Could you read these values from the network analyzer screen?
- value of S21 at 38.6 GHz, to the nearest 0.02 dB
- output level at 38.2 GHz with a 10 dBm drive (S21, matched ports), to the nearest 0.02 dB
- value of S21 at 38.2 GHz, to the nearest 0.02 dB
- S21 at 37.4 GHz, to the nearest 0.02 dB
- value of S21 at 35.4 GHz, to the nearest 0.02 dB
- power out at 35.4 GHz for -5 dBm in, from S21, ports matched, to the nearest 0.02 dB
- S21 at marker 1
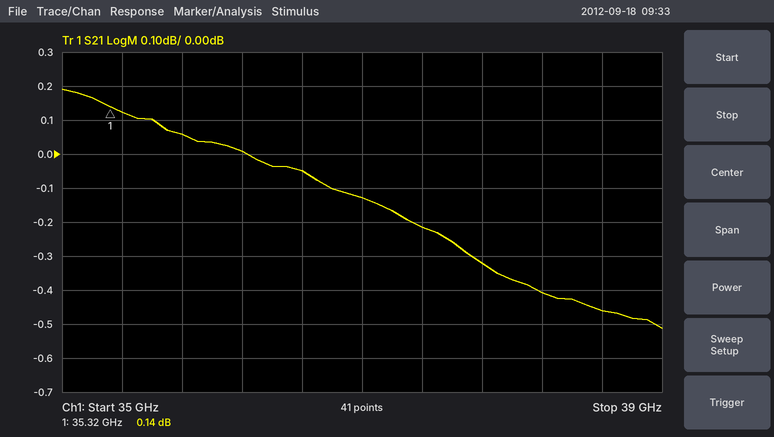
-0.46 dB
9.60 dBm
-0.40 dB
-0.22 dB
0.12 dB
-4.88 dBm
0.14 dB
